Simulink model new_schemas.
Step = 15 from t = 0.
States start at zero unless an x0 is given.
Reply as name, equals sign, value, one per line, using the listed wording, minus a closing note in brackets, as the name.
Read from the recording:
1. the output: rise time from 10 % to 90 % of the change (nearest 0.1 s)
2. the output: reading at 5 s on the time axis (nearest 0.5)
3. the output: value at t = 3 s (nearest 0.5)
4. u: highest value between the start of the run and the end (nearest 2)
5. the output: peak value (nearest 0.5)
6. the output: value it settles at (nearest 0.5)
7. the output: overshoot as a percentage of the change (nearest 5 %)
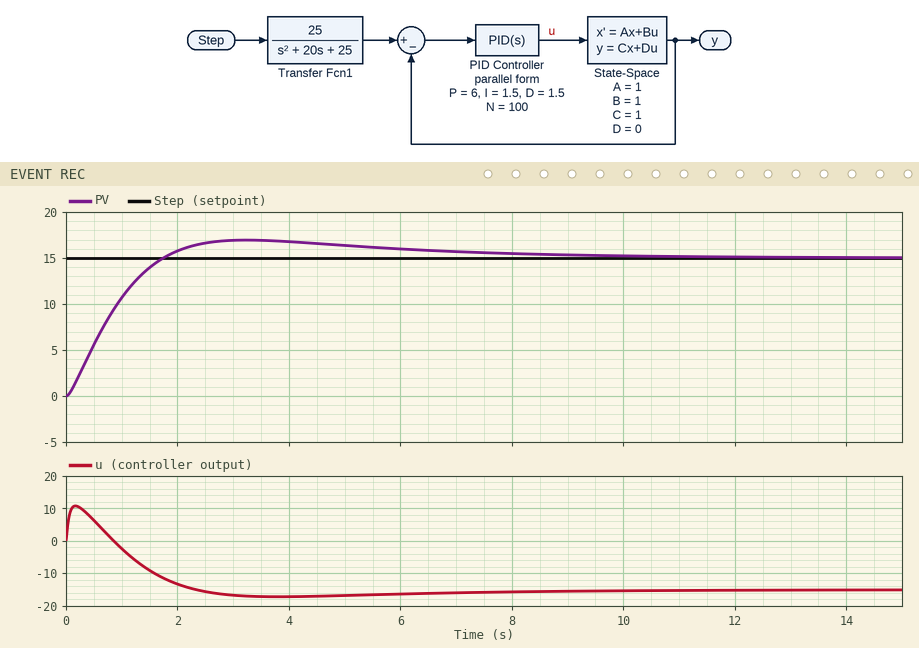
the output: rise time from 10 % to 90 % of the change = 1.2 s
the output: reading at 5 s on the time axis = 16.5
the output: value at t = 3 s = 17.0
u: highest value between the start of the run and the end = 10
the output: peak value = 17.0
the output: value it settles at = 15.0
the output: overshoot as a percentage of the change = 15 %
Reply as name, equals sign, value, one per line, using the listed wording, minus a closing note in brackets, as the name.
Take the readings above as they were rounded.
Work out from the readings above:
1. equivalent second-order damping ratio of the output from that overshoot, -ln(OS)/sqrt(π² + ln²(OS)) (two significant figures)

equivalent second-order damping ratio of the output from that overshoot, -ln(OS)/sqrt(π² + ln²(OS)) = 0.52
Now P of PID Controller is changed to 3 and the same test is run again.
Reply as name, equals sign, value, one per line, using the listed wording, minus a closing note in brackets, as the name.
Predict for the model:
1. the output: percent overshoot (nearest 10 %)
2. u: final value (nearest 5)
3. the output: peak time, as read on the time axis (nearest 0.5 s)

the output: percent overshoot = 30 %
u: final value = -15
the output: peak time, as read on the time axis = 3.0 s
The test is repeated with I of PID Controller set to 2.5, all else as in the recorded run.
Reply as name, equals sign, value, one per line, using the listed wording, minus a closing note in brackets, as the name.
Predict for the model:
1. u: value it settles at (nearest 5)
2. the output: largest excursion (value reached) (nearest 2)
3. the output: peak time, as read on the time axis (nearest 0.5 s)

u: value it settles at = -15
the output: largest excursion (value reached) = 16
the output: peak time, as read on the time axis = 3.0 s
